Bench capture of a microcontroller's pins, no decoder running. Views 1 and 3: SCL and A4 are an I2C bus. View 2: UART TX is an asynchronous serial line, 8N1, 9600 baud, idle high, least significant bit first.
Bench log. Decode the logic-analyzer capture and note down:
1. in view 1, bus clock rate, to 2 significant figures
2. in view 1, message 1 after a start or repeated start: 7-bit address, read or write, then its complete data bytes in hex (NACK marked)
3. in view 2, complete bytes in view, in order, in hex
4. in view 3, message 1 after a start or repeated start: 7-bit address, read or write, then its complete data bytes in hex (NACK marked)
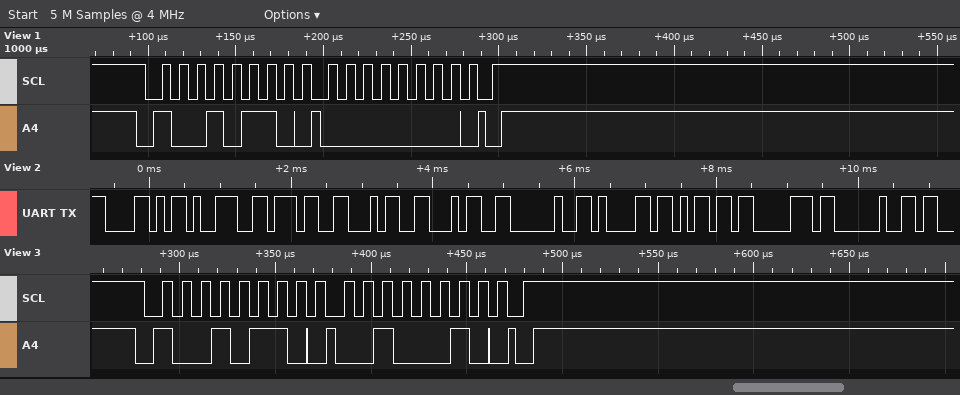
100 kHz
0x4B write: 00
58 39 37 34 34 20 61 6D 70 20
0x4B write: 22
